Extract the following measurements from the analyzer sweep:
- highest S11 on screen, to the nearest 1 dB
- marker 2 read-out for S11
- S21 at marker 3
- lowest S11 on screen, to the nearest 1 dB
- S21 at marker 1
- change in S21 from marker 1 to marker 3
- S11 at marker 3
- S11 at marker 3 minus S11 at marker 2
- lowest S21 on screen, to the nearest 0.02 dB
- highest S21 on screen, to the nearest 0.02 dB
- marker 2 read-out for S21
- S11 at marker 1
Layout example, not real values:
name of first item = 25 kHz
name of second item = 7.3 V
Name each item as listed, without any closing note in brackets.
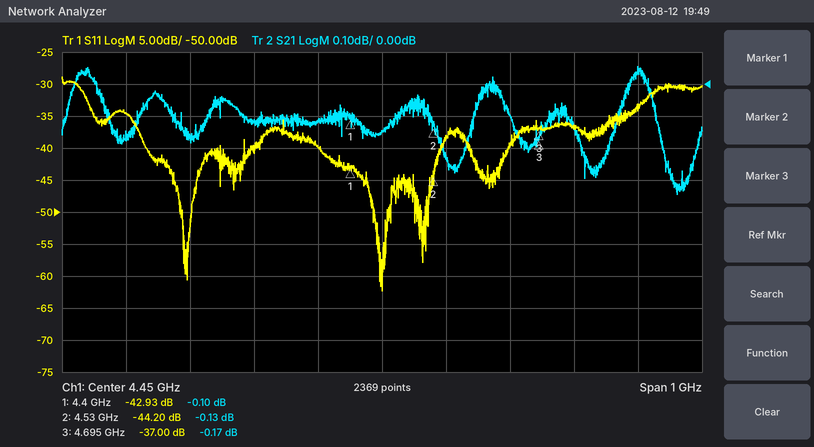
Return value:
highest S11 on screen, to the nearest 1 dB = -29 dB
marker 2 read-out for S11 = -44.20 dB
S21 at marker 3 = -0.17 dB
lowest S11 on screen, to the nearest 1 dB = -62 dB
S21 at marker 1 = -0.10 dB
change in S21 from marker 1 to marker 3 = -0.07 dB
S11 at marker 3 = -37.00 dB
S11 at marker 3 minus S11 at marker 2 = 7.20 dB
lowest S21 on screen, to the nearest 0.02 dB = -0.34 dB
highest S21 on screen, to the nearest 0.02 dB = 0.06 dB
marker 2 read-out for S21 = -0.13 dB
S11 at marker 1 = -42.93 dB
